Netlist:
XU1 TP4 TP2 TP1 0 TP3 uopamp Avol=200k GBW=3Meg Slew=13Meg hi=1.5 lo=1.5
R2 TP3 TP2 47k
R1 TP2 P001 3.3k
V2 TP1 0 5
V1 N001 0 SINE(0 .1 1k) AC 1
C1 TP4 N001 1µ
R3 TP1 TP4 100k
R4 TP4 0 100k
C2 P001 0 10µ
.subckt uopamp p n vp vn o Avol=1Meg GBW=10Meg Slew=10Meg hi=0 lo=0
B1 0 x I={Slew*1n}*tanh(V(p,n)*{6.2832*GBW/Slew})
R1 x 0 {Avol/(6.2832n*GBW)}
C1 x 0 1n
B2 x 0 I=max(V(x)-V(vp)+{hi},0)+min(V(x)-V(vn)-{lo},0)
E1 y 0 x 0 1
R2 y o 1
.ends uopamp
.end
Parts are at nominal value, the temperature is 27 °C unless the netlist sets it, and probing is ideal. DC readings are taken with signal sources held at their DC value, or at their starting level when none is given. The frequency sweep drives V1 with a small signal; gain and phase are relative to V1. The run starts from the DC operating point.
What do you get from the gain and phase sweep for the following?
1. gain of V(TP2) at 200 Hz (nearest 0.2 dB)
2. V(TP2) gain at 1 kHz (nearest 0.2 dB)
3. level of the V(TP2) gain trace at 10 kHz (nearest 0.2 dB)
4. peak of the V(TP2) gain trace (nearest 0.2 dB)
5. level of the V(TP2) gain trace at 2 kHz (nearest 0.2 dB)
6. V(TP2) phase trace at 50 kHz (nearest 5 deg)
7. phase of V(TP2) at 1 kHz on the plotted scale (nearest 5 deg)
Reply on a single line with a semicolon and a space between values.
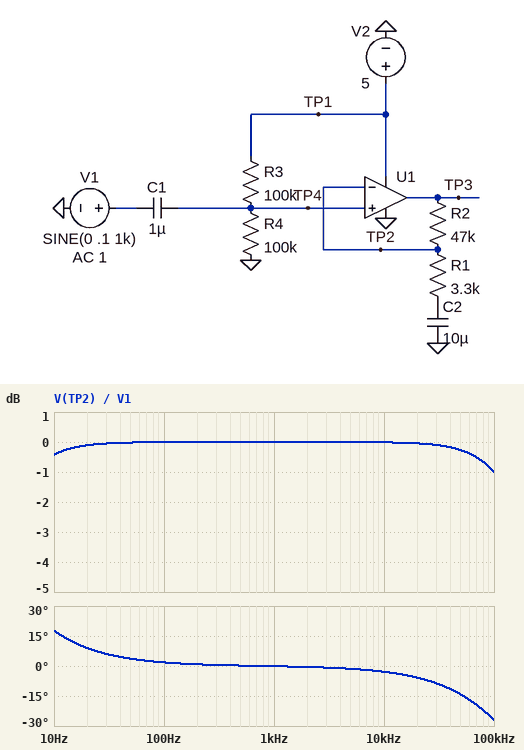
0 dB; 0 dB; 0 dB; 0 dB; 0 dB; -15 deg; 0 deg
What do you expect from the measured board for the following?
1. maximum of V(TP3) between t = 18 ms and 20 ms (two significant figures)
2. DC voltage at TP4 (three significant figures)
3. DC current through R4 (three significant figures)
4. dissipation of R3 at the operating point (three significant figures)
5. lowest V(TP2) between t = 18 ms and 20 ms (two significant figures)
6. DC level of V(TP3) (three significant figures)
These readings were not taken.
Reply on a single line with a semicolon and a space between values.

3.5 V; 2.50 V; 25.0 µA; 62.5 µW; 2.4 V; 2.50 V
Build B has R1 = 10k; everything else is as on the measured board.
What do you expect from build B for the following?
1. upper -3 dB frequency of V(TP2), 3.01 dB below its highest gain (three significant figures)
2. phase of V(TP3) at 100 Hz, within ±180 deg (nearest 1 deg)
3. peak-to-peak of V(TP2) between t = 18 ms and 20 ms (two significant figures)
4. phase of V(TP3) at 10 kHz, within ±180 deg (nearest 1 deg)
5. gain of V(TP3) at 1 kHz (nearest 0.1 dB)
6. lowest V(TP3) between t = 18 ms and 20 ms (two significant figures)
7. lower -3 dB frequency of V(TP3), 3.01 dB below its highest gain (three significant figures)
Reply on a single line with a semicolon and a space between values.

526 kHz; 3 deg; 200 mV; -1 deg; 15.1 dB; 1.9 V; 3.78 Hz
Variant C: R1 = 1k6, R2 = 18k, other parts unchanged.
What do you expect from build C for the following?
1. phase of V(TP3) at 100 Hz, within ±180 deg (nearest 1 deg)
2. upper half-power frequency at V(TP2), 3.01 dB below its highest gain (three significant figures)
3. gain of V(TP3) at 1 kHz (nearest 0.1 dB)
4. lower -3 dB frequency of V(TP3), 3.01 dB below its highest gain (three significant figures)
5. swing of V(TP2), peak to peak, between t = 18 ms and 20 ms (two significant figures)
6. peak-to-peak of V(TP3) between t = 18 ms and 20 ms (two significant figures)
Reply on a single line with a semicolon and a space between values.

7 deg; 245 kHz; 21.8 dB; 10.8 Hz; 160 mV; 2.0 V
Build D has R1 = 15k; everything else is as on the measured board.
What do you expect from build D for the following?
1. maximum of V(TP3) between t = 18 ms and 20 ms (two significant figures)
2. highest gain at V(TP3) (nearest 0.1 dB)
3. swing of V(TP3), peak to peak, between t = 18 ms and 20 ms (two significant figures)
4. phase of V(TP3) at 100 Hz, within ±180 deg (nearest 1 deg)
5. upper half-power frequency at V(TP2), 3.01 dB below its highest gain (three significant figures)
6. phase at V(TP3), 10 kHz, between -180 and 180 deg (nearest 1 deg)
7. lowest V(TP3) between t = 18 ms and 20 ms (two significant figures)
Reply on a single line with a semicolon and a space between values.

2.9 V; 12.3 dB; 830 mV; 2 deg; 726 kHz; -1 deg; 2.1 V
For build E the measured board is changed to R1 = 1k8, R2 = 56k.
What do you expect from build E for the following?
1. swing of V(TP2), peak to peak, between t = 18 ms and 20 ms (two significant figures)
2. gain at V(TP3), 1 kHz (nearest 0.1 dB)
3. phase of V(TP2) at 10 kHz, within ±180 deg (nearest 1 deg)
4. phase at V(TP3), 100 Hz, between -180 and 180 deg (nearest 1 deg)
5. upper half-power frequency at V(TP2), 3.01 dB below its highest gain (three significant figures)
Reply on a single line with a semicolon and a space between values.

63 mV; 30.1 dB; -6 deg; 7 deg; 93.4 kHz
